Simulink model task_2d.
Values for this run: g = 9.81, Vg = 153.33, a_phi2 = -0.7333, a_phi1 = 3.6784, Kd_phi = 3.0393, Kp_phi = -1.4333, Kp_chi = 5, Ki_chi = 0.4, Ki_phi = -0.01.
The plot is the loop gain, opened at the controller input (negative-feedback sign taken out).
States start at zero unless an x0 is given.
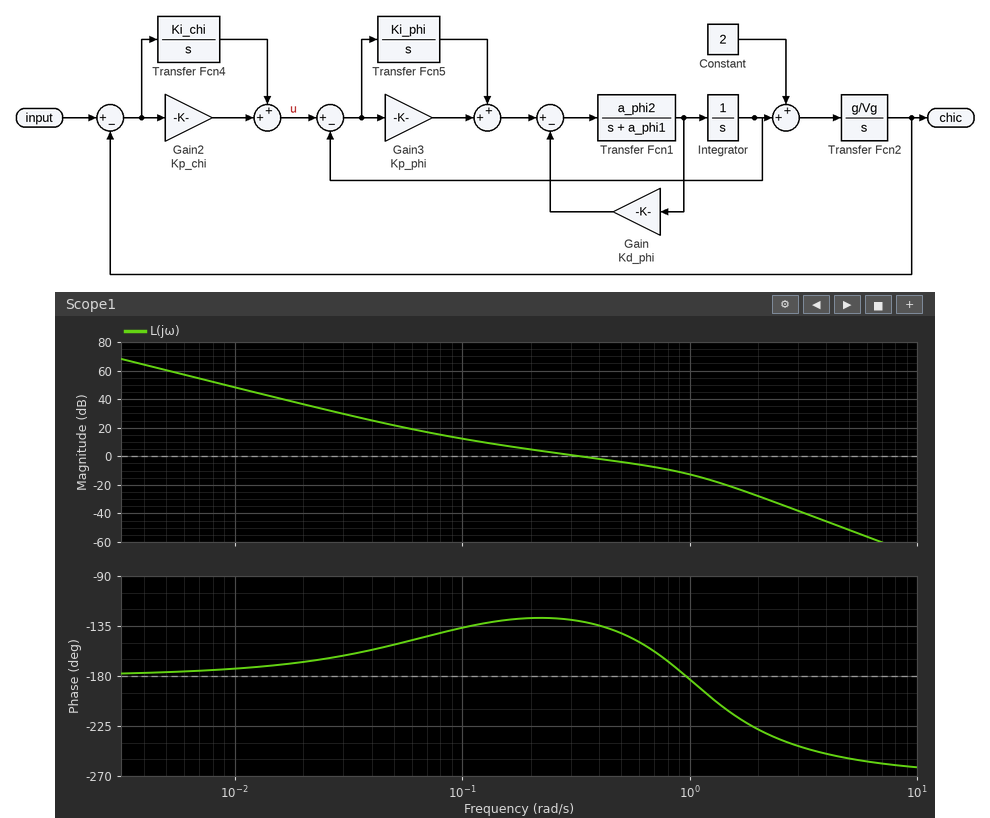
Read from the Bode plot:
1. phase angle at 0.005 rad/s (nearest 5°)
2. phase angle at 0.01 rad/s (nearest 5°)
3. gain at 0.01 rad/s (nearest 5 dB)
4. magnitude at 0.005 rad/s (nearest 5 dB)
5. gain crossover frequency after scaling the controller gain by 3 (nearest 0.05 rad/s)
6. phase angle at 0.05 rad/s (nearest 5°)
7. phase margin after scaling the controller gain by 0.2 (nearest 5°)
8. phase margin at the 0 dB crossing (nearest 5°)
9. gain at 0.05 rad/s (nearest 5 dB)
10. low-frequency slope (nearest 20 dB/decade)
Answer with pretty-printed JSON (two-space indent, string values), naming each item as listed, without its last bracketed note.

{
  "phase angle at 0.005 rad/s": "-175°",
  "phase angle at 0.01 rad/s": "-175°",
  "gain at 0.01 rad/s": "50 dB",
  "magnitude at 0.005 rad/s": "60 dB",
  "gain crossover frequency after scaling the controller gain by 3": "0.80 rad/s",
  "phase angle at 0.05 rad/s": "-150°",
  "phase margin after scaling the controller gain by 0.2": "40°",
  "phase margin at the 0 dB crossing": "50°",
  "gain at 0.05 rad/s": "20 dB",
  "low-frequency slope": "-40 dB/decade"
}
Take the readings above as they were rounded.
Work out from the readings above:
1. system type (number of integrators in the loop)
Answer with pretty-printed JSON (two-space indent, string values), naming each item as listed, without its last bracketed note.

{
  "system type": "2"
}
